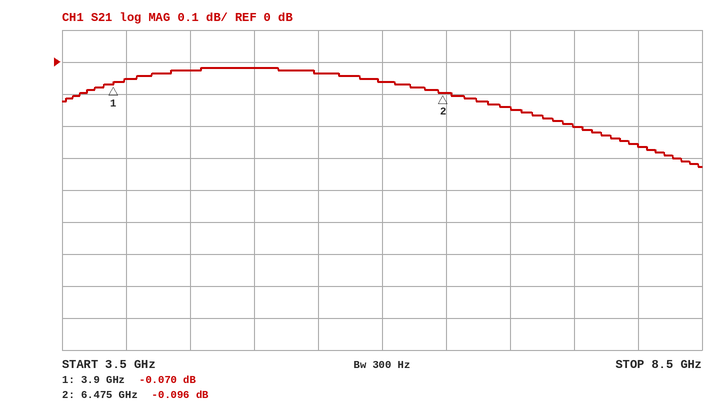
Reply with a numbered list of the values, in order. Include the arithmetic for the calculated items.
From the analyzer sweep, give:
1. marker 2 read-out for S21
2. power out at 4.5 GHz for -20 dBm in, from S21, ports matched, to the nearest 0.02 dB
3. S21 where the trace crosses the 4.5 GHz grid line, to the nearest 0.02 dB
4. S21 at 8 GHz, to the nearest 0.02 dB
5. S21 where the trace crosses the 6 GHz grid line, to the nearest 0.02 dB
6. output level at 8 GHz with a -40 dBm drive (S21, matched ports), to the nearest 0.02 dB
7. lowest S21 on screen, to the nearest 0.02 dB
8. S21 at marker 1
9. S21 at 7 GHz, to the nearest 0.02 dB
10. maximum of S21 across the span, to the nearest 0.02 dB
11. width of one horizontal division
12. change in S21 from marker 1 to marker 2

1. -0.096 dB
2. -20 dBm + (-0.02 dB) = -20.02 dBm
3. -0.02 dB
4. -0.26 dB
5. -0.06 dB
6. -40 dBm + (-0.26 dB) = -40.26 dBm
7. -0.32 dB
8. -0.070 dB
9. -0.14 dB
10. -0.02 dB
11. 500 MHz
12. -0.096 − (-0.07) = -0.026 dB
